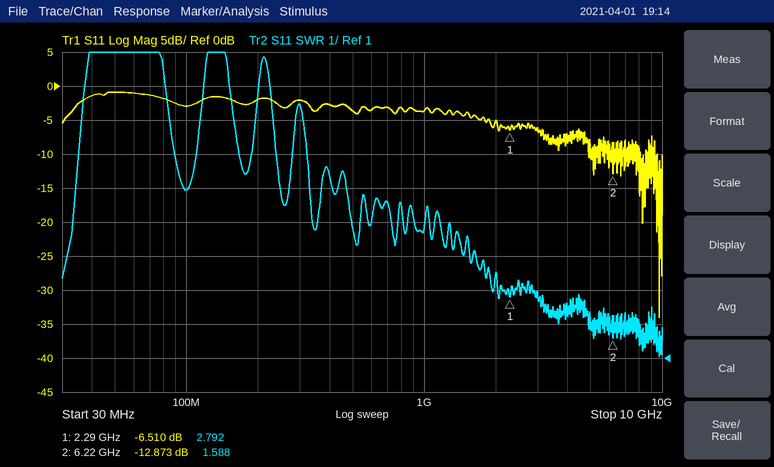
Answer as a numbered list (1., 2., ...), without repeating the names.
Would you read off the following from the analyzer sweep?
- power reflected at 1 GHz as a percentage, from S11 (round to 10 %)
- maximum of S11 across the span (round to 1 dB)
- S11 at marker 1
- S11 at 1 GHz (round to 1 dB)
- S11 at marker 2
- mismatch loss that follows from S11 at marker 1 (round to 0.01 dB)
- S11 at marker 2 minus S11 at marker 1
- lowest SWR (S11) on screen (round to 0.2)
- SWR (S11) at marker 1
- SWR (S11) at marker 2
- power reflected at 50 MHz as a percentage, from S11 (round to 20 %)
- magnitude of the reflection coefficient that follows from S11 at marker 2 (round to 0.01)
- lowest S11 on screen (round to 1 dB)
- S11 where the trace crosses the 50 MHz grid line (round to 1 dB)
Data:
1. 40 %
2. -1 dB
3. -6.510 dB
4. -4 dB
5. -12.873 dB
6. 1.10 dB
7. -6.363 dB
8. 1.0
9. 2.792
10. 1.588
11. 80 %
12. 0.23
13. -34 dB
14. -1 dB
